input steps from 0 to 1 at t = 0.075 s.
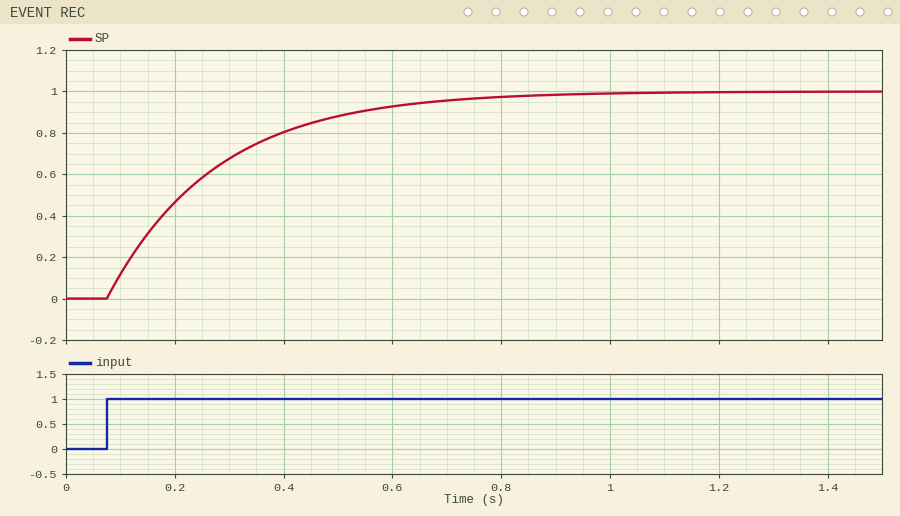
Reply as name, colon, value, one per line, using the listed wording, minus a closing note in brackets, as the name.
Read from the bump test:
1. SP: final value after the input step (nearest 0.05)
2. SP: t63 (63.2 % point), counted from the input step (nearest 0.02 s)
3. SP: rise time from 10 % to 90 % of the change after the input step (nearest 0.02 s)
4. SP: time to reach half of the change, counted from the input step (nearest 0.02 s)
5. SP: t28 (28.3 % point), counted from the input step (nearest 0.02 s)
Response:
SP: final value after the input step: 1.00
SP: t63 (63.2 % point), counted from the input step: 0.20 s
SP: rise time from 10 % to 90 % of the change after the input step: 0.44 s
SP: time to reach half of the change, counted from the input step: 0.14 s
SP: t28 (28.3 % point), counted from the input step: 0.06 s
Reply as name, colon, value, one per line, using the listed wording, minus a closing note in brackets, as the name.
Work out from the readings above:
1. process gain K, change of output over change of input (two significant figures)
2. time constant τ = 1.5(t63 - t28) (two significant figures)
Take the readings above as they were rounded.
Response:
process gain K, change of output over change of input: 1.0
time constant τ = 1.5(t63 - t28): 0.21 s
